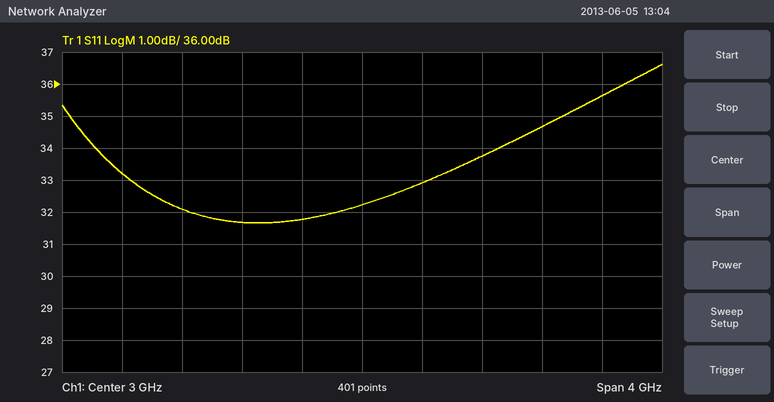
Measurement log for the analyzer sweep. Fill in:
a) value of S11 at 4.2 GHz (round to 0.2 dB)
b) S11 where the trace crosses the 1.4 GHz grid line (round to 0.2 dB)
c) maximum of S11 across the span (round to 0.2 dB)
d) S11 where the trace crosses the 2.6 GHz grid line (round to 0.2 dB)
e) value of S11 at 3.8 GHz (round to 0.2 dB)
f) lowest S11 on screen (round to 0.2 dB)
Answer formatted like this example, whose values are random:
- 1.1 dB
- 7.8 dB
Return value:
- 34.6 dB
- 33.2 dB
- 36.6 dB
- 31.8 dB
- 33.8 dB
- 31.6 dB
